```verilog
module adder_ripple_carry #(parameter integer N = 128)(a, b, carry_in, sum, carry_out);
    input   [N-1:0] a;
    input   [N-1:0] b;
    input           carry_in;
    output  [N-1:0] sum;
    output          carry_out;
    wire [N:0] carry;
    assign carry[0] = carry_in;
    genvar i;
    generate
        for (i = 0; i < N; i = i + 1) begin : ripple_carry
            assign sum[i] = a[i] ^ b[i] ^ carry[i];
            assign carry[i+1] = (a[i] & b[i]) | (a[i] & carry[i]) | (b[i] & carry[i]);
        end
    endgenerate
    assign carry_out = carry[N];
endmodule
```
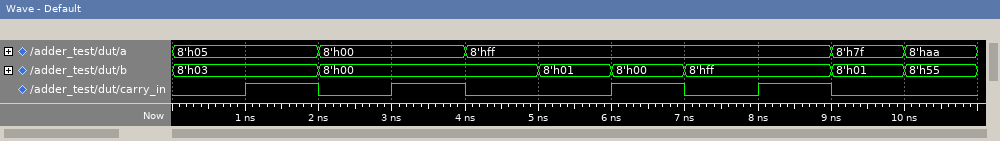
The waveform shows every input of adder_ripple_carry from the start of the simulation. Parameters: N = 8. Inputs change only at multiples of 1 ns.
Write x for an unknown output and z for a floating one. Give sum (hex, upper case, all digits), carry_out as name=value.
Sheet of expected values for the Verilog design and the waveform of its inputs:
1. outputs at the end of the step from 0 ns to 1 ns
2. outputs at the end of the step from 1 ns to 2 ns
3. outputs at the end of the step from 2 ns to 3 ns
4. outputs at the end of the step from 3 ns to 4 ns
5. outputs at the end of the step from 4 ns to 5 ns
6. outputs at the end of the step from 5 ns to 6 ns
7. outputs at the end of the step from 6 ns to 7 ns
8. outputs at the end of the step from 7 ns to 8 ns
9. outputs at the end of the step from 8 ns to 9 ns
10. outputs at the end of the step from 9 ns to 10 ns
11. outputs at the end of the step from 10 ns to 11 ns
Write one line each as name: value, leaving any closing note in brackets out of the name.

outputs at the end of the step from 0 ns to 1 ns: sum=08, carry_out=0
outputs at the end of the step from 1 ns to 2 ns: sum=09, carry_out=0
outputs at the end of the step from 2 ns to 3 ns: sum=00, carry_out=0
outputs at the end of the step from 3 ns to 4 ns: sum=01, carry_out=0
outputs at the end of the step from 4 ns to 5 ns: sum=FF, carry_out=0
outputs at the end of the step from 5 ns to 6 ns: sum=00, carry_out=1
outputs at the end of the step from 6 ns to 7 ns: sum=00, carry_out=1
outputs at the end of the step from 7 ns to 8 ns: sum=FE, carry_out=1
outputs at the end of the step from 8 ns to 9 ns: sum=FF, carry_out=1
outputs at the end of the step from 9 ns to 10 ns: sum=80, carry_out=0
outputs at the end of the step from 10 ns to 11 ns: sum=FF, carry_out=0
